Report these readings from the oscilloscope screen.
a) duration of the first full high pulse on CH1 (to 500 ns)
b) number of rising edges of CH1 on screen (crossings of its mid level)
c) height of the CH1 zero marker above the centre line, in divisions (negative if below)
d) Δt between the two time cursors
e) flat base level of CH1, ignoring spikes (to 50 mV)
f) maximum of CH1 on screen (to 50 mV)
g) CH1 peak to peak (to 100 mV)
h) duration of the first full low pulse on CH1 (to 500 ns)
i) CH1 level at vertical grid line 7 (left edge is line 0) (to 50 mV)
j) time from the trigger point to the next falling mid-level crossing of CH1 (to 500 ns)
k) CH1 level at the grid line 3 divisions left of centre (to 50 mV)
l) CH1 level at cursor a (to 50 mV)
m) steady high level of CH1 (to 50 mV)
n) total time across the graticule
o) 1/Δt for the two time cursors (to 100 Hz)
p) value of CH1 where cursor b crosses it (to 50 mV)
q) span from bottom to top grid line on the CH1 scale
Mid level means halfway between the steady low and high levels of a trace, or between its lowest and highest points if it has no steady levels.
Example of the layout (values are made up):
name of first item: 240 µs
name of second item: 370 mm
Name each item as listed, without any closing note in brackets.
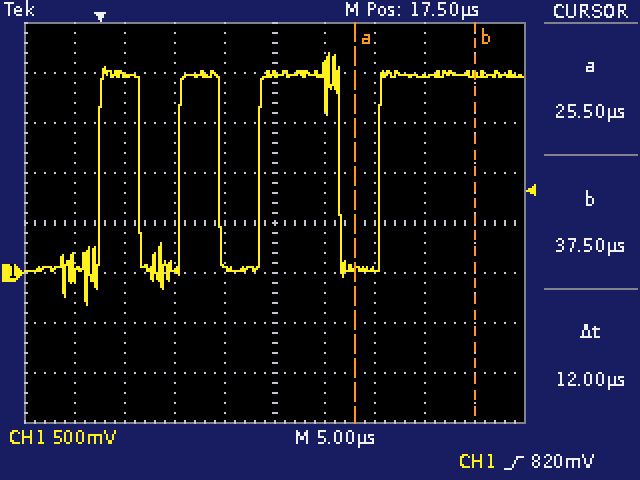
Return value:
duration of the first full high pulse on CH1: 4.0 µs
number of rising edges of CH1 on screen: 4
height of the CH1 zero marker above the centre line, in divisions: -1.0 div
Δt between the two time cursors: 12 µs
flat base level of CH1, ignoring spikes: 50 mV
maximum of CH1 on screen: 2.20 V
CH1 peak to peak: 2.50 V
duration of the first full low pulse on CH1: 4.0 µs
CH1 level at vertical grid line 7 (left edge is line 0): 50 mV
time from the trigger point to the next falling mid-level crossing of CH1: 4.0 µs
CH1 level at the grid line 3 divisions left of centre: 2.00 V
CH1 level at cursor a: 50 mV
steady high level of CH1: 2.00 V
total time across the graticule: 50 µs
1/Δt for the two time cursors: 83.3 kHz
value of CH1 where cursor b crosses it: 2.00 V
span from bottom to top grid line on the CH1 scale: 4 V
